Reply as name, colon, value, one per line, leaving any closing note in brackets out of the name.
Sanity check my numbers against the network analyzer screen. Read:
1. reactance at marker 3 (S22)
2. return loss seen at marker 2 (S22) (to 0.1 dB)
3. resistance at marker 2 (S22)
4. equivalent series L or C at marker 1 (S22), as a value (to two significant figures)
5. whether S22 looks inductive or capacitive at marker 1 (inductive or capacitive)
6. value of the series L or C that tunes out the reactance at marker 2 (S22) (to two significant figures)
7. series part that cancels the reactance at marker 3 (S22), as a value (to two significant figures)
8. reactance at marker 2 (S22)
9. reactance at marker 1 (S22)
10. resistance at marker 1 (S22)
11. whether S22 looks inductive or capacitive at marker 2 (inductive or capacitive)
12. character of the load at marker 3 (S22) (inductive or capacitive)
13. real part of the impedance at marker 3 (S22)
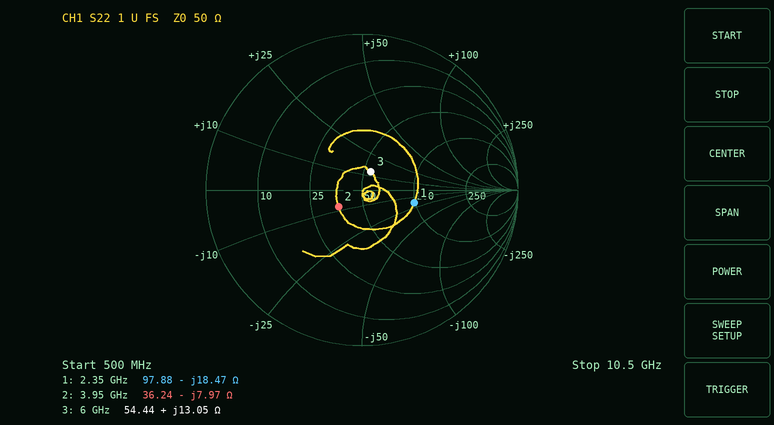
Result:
reactance at marker 3: +13.05 Ω
return loss seen at marker 2 (S22): 14.7 dB
resistance at marker 2: 36.24 Ω
equivalent series L or C at marker 1 (S22), as a value: 3.7 pF
whether S22 looks inductive or capacitive at marker 1: capacitive
value of the series L or C that tunes out the reactance at marker 2 (S22): 320 pH
series part that cancels the reactance at marker 3 (S22), as a value: 2.0 pF
reactance at marker 2: -7.97 Ω
reactance at marker 1: -18.47 Ω
resistance at marker 1: 97.88 Ω
whether S22 looks inductive or capacitive at marker 2: capacitive
character of the load at marker 3 (S22): inductive
real part of the impedance at marker 3: 54.44 Ω
